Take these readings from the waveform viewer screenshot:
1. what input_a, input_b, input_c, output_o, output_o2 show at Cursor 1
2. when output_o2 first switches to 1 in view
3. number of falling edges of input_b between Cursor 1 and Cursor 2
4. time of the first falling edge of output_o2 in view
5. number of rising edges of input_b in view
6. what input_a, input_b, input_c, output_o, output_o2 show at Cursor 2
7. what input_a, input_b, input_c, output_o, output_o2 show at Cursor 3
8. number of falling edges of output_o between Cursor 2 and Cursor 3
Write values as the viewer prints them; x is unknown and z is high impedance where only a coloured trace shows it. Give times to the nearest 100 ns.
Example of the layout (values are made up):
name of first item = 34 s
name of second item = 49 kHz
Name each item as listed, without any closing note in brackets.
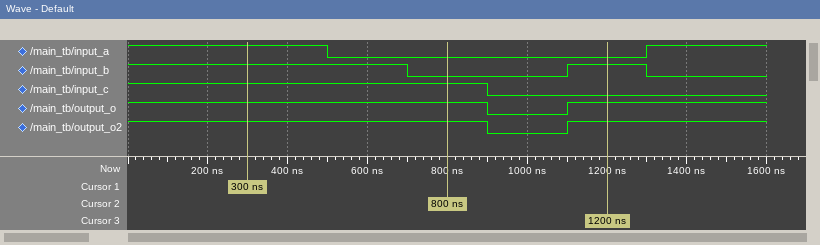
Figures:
what input_a, input_b, input_c, output_o, output_o2 show at Cursor 1 = input_a=1, input_b=1, input_c=1, output_o=1, output_o2=1
when output_o2 first switches to 1 in view = 1100 ns
number of falling edges of input_b between Cursor 1 and Cursor 2 = 1
time of the first falling edge of output_o2 in view = 900 ns
number of rising edges of input_b in view = 1
what input_a, input_b, input_c, output_o, output_o2 show at Cursor 2 = input_a=0, input_b=0, input_c=1, output_o=1, output_o2=1
what input_a, input_b, input_c, output_o, output_o2 show at Cursor 3 = input_a=0, input_b=1, input_c=0, output_o=1, output_o2=1
number of falling edges of output_o between Cursor 2 and Cursor 3 = 1
